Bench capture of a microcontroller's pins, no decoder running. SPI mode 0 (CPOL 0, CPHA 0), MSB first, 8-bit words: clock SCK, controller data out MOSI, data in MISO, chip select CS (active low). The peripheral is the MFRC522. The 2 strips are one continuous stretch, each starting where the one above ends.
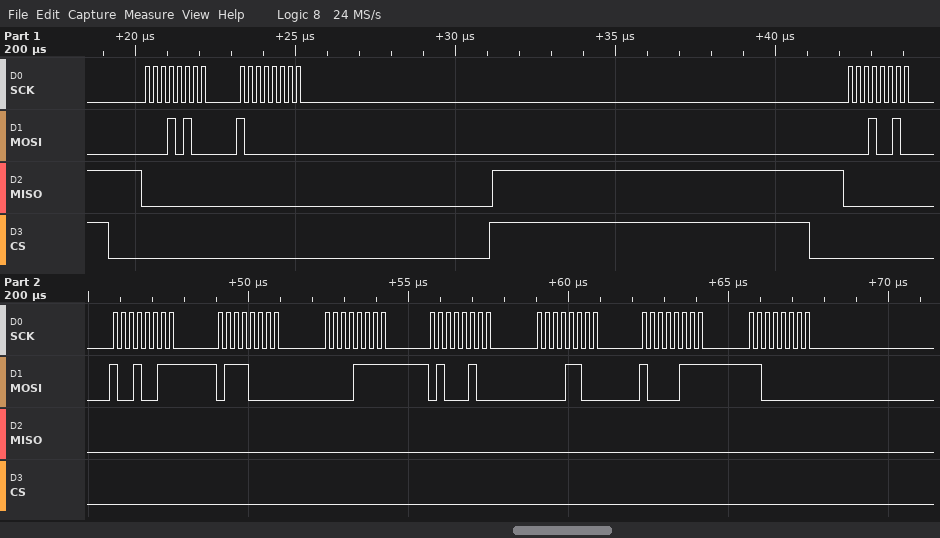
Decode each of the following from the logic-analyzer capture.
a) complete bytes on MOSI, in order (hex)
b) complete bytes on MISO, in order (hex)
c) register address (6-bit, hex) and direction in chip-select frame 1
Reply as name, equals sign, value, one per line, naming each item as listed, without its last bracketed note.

complete bytes on MOSI, in order = 14 80 12 93 70 0F 44 0C 87 C0
complete bytes on MISO, in order = 00 00 00 00 00 00 00 00 00 00
register address (6-bit, hex) and direction in chip-select frame 1 = 0x0A write
